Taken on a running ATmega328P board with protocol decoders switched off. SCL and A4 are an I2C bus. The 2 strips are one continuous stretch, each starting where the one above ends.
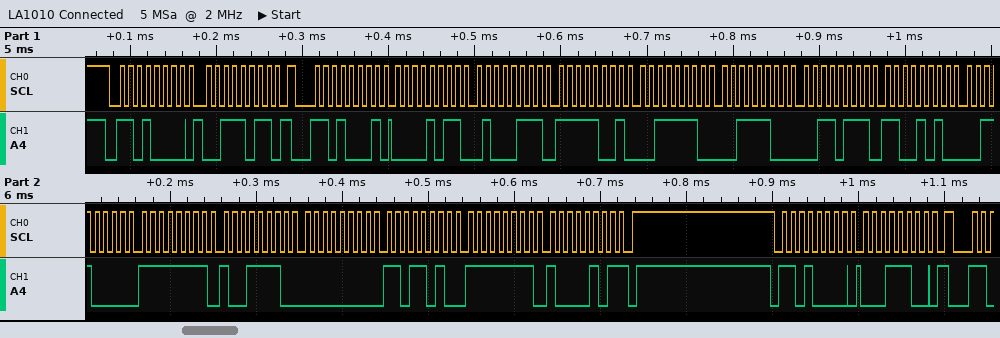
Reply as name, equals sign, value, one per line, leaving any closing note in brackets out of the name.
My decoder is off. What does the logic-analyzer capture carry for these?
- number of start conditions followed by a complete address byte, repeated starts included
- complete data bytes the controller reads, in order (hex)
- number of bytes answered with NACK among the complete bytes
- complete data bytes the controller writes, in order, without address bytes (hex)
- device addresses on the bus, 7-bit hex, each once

number of start conditions followed by a complete address byte, repeated starts included = 3
complete data bytes the controller reads, in order = 0B 47 F9 3E 3C 37 CA 30 FF 9E 00 DA FF 85
number of bytes answered with NACK among the complete bytes = 1
complete data bytes the controller writes, in order, without address bytes = 3B 1C
device addresses on the bus, 7-bit hex, each once = 0x68
